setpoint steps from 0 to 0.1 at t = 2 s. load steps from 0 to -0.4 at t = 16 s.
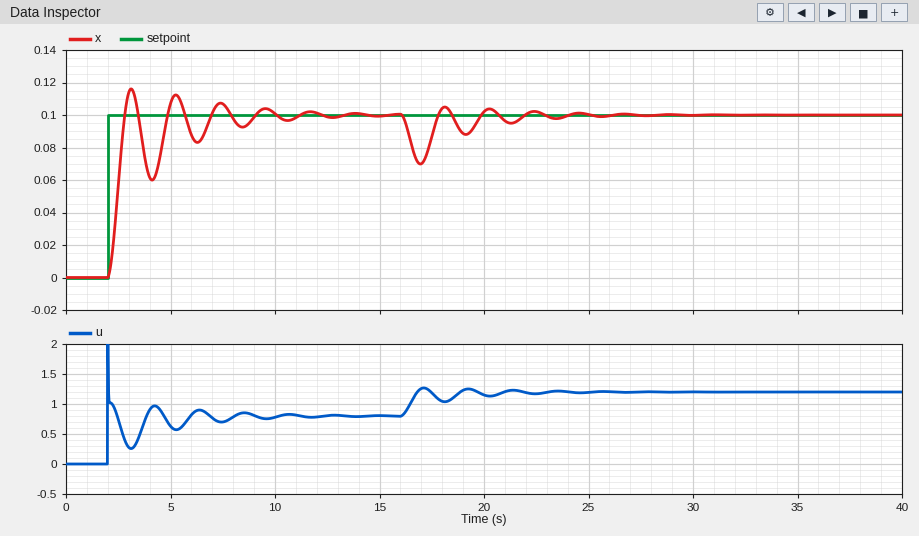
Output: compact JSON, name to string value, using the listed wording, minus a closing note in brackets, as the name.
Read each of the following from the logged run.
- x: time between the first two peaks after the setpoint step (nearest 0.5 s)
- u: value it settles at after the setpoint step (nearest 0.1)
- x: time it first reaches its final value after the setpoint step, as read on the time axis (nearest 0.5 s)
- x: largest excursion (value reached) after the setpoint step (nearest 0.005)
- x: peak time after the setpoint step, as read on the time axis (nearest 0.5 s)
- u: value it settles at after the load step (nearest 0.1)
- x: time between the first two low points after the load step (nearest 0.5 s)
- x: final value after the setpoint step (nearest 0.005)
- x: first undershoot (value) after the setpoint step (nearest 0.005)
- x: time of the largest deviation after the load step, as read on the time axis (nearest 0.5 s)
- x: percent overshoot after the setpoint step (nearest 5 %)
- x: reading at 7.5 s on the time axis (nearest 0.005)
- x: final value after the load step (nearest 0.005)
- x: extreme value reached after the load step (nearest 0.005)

{"x: time between the first two peaks after the setpoint step": "2.0 s", "u: value it settles at after the setpoint step": "0.8", "x: time it first reaches its final value after the setpoint step, as read on the time axis": "3.0 s", "x: largest excursion (value reached) after the setpoint step": "0.115", "x: peak time after the setpoint step, as read on the time axis": "3.0 s", "u: value it settles at after the load step": "1.2", "x: time between the first two low points after the load step": "2.0 s", "x: final value after the setpoint step": "0.100", "x: first undershoot (value) after the setpoint step": "0.060", "x: time of the largest deviation after the load step, as read on the time axis": "17.0 s", "x: percent overshoot after the setpoint step": "15 %", "x: reading at 7.5 s on the time axis": "0.105", "x: final value after the load step": "0.100", "x: extreme value reached after the load step": "0.070"}
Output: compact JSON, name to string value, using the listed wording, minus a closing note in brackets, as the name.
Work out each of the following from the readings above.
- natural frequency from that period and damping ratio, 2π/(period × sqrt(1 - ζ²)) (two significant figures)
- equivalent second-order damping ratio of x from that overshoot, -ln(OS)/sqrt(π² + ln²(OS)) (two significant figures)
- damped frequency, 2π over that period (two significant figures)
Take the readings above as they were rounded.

{"natural frequency from that period and damping ratio, 2π/(period × sqrt(1 - ζ²))": "3.7 rad/s", "equivalent second-order damping ratio of x from that overshoot, -ln(OS)/sqrt(π² + ln²(OS))": "0.52", "damped frequency, 2π over that period": "3.1 rad/s"}
